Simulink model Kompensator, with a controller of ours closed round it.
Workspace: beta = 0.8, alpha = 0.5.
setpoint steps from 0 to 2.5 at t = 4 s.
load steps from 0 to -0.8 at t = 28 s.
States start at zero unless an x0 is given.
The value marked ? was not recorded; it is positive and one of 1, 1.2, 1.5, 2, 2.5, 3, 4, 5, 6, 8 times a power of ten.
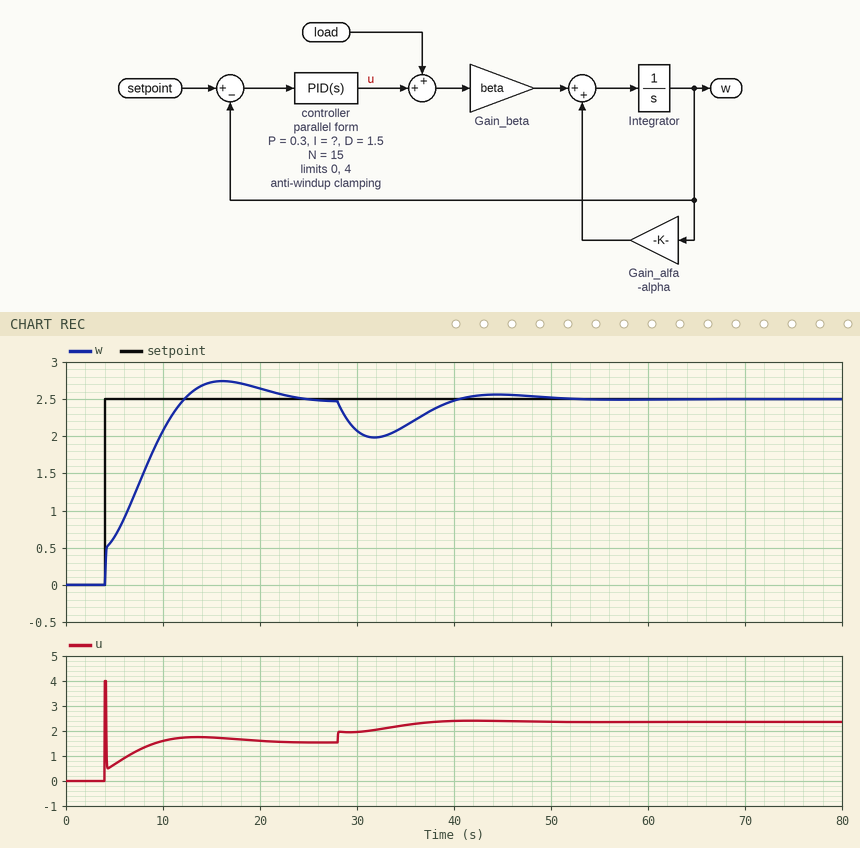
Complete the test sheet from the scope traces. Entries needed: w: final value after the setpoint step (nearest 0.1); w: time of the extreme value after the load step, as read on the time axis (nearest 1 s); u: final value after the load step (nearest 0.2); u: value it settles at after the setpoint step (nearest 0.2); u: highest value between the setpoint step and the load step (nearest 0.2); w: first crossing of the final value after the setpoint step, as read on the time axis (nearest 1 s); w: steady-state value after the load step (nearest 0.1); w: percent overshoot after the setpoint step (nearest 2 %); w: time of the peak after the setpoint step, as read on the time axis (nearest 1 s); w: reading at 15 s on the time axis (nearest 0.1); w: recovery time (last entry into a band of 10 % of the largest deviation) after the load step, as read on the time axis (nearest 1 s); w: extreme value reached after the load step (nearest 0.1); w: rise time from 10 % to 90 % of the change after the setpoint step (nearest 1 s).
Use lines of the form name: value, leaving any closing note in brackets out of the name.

w: final value after the setpoint step: 2.5
w: time of the extreme value after the load step, as read on the time axis: 32 s
u: final value after the load step: 2.4
u: value it settles at after the setpoint step: 1.6
u: highest value between the setpoint step and the load step: 4.0
w: first crossing of the final value after the setpoint step, as read on the time axis: 12 s
w: steady-state value after the load step: 2.5
w: percent overshoot after the setpoint step: 10 %
w: time of the peak after the setpoint step, as read on the time axis: 16 s
w: reading at 15 s on the time axis: 2.7
w: recovery time (last entry into a band of 10 % of the largest deviation) after the load step, as read on the time axis: 47 s
w: extreme value reached after the load step: 2.0
w: rise time from 10 % to 90 % of the change after the setpoint step: 7 s
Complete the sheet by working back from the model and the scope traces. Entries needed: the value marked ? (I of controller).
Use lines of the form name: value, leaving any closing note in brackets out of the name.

the value marked ?: 0.25
